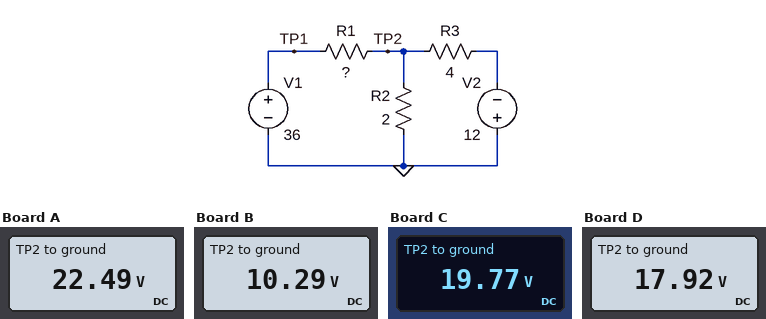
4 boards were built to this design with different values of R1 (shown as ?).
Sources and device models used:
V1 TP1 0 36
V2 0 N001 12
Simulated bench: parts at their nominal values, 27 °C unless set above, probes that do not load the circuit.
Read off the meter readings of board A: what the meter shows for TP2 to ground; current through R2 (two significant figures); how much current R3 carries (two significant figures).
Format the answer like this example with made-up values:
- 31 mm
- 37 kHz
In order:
- 22.49 V
- 11 A
- 8.6 A
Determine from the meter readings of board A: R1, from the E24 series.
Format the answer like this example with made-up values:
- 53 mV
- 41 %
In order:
- 0.68 Ω
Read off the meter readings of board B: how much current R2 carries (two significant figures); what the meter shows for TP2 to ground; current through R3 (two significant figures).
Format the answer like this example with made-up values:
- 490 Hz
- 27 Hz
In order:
- 5.1 A
- 10.29 V
- 5.6 A
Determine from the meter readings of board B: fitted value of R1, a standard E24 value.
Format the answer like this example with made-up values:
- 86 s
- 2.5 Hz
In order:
- 2.4 Ω
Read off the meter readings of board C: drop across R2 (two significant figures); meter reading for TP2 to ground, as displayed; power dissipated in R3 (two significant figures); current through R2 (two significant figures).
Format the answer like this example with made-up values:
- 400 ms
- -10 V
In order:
- 20 V
- 19.77 V
- 250 W
- 9.9 A
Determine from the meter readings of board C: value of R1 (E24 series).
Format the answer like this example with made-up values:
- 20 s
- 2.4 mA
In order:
- 0.91 Ω
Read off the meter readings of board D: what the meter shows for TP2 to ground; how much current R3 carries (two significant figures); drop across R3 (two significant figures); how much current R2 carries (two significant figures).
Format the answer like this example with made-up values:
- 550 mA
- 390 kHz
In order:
- 17.92 V
- 7.5 A
- 30 V
- 9.0 A
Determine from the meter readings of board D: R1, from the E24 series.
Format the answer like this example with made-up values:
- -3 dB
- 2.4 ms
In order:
- 1.1 Ω
